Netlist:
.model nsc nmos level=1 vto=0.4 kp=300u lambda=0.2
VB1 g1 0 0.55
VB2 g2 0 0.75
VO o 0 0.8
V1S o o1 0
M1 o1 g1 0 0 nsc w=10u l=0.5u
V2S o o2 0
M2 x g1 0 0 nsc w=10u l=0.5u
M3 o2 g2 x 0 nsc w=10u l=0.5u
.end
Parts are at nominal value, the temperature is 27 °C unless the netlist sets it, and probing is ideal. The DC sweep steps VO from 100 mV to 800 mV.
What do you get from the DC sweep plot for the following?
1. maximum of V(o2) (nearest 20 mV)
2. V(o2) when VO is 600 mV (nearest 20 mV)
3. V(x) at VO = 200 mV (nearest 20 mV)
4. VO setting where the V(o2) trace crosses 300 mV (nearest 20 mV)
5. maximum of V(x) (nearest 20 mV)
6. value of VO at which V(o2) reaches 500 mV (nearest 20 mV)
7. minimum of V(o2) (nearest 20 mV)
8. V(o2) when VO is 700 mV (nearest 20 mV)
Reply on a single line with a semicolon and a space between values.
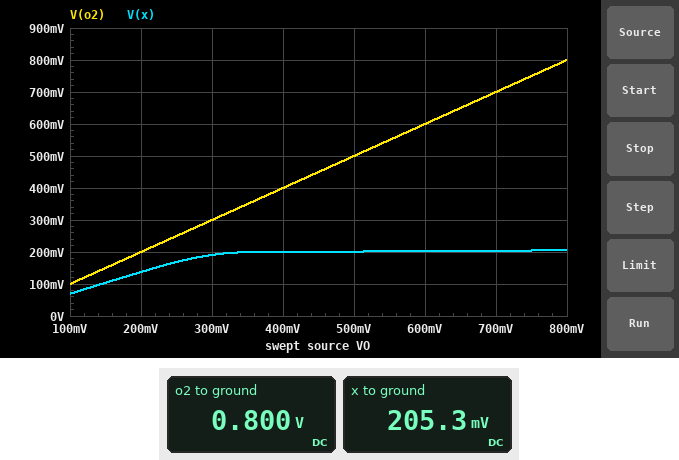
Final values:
800 mV; 600 mV; 140 mV; 300 mV; 200 mV; 500 mV; 100 mV; 700 mV
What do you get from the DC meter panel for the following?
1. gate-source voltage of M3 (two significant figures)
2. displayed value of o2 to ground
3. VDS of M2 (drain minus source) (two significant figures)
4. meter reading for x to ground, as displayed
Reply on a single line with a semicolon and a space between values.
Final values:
540 mV; 0.800 V; 210 mV; 205.3 mV
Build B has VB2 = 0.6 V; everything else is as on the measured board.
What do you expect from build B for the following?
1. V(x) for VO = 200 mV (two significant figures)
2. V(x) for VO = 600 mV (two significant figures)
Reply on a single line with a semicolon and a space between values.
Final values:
72 mV; 75 mV
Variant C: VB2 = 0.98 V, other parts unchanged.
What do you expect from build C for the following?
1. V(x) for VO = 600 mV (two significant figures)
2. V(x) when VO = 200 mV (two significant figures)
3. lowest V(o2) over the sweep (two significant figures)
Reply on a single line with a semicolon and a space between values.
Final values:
430 mV; 170 mV; 100 mV
